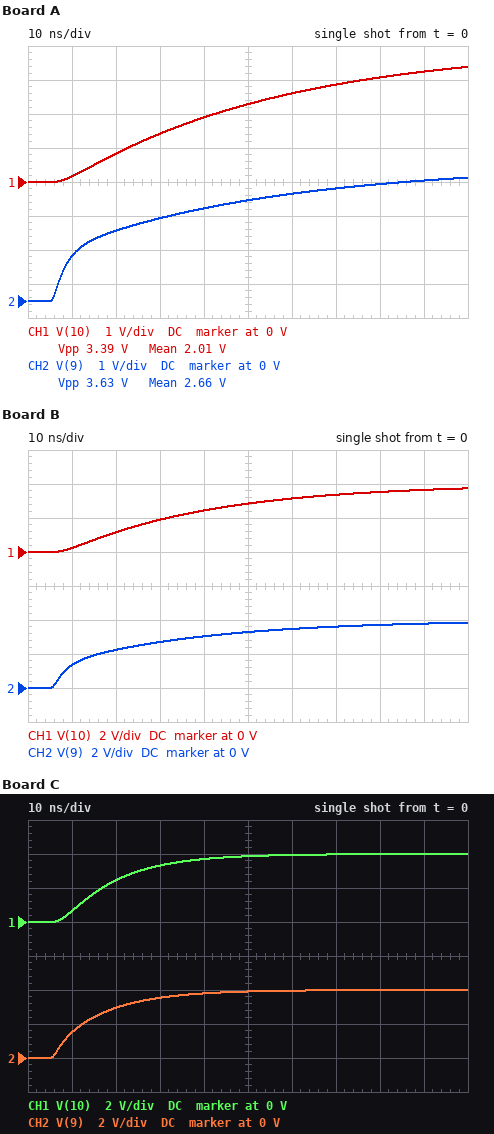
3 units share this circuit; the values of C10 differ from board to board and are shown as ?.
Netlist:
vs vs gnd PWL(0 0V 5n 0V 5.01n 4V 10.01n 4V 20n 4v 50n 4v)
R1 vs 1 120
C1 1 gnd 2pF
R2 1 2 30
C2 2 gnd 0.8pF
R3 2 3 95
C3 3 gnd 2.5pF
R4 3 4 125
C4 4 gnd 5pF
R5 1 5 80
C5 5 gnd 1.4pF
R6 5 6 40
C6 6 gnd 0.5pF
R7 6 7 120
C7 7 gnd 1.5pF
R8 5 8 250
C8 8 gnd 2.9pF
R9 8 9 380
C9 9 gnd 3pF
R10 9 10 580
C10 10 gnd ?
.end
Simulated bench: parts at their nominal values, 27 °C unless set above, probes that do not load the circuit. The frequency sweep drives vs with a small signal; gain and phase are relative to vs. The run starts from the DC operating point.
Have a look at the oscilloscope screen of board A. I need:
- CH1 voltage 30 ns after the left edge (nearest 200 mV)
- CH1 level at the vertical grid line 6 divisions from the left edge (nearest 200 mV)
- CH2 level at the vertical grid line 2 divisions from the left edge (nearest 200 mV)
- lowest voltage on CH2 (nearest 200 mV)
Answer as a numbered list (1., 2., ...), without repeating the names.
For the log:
1. 1.4 V
2. 2.6 V
3. 2.0 V
4. 0 V
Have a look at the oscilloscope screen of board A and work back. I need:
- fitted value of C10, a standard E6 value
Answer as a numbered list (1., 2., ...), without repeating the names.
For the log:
1. 33 pF
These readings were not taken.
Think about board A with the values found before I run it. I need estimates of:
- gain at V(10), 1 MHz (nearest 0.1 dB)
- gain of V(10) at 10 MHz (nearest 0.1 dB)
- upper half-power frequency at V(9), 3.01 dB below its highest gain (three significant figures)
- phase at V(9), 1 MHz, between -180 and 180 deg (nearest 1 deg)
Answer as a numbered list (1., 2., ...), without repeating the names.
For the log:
1. -0.4 dB
2. -10.3 dB
3. 3.91 MHz
4. -11 deg
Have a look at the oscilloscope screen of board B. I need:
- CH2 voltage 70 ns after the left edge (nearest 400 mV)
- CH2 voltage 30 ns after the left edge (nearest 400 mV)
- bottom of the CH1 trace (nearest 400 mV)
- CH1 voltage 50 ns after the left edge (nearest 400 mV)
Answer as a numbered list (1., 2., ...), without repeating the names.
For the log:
1. 3.6 V
2. 2.8 V
3. 0 V
4. 2.8 V
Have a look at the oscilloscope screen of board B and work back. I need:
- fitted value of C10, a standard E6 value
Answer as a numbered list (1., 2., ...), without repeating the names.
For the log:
1. 22 pF
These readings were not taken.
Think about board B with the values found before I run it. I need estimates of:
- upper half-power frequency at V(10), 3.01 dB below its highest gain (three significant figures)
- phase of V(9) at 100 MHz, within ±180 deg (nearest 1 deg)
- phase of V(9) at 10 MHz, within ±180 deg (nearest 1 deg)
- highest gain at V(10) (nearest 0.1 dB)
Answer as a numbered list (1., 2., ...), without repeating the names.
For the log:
1. 4.76 MHz
2. -92 deg
3. -38 deg
4. 0 dB
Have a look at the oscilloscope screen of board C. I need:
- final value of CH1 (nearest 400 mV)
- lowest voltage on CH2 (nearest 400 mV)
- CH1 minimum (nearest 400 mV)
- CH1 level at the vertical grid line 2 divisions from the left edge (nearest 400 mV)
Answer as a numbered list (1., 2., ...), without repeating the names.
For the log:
1. 4.0 V
2. 0 V
3. 0 V
4. 2.4 V
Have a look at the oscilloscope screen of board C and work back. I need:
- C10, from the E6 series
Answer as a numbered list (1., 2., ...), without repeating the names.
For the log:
1. 6.8 pF
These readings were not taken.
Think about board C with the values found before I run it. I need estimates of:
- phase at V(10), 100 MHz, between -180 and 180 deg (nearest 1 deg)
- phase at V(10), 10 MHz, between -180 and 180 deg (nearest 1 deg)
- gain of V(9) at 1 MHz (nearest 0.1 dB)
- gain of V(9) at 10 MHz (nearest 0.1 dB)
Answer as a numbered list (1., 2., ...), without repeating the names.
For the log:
1. -166 deg
2. -49 deg
3. 0 dB
4. -1.8 dB
